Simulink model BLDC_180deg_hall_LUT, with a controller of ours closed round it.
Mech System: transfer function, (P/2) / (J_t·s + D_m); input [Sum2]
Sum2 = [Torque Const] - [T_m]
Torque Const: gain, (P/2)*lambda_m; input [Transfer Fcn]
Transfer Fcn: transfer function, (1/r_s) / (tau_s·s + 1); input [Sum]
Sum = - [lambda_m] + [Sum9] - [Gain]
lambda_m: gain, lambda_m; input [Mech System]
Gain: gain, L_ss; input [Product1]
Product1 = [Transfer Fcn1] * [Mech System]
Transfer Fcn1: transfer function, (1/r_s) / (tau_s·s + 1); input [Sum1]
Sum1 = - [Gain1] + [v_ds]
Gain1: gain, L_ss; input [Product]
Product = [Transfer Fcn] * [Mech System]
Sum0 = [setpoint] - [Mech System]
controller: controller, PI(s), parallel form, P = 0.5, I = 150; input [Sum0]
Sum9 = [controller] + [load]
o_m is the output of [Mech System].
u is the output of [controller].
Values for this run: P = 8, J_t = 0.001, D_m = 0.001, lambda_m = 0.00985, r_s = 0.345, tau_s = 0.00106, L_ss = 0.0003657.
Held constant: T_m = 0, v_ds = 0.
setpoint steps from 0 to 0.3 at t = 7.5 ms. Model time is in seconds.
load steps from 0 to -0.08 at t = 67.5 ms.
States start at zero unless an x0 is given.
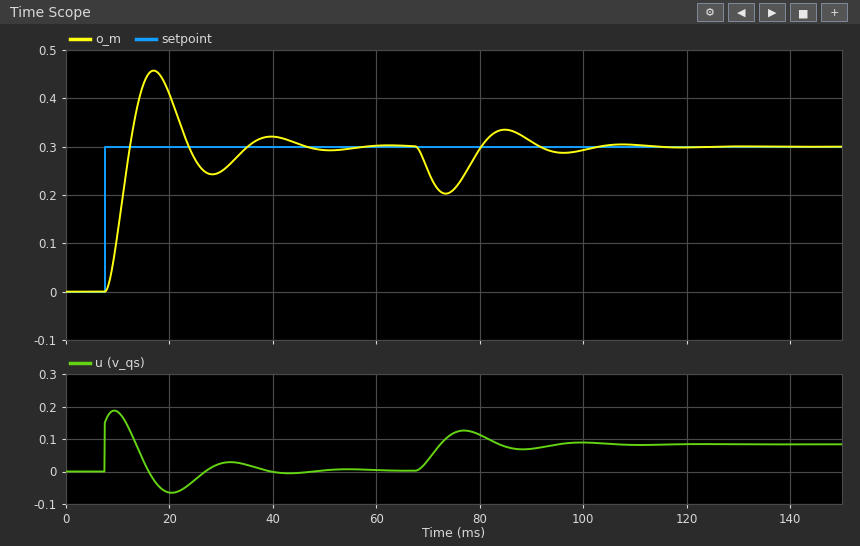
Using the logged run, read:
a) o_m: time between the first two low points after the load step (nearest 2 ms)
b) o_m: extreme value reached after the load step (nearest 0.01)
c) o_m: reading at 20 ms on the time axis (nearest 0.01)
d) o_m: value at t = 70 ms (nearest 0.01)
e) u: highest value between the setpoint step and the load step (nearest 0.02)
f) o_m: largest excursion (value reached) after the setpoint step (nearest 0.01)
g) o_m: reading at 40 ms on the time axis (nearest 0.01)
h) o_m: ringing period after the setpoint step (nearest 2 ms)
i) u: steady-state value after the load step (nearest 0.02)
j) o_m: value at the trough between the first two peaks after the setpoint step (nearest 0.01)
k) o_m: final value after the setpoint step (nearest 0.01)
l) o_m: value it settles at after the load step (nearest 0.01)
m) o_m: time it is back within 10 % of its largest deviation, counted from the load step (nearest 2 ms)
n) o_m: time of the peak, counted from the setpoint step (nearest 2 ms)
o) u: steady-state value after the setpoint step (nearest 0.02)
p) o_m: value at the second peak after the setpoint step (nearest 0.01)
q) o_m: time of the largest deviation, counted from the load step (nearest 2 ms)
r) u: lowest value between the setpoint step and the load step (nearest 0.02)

22 ms
0.20
0.41
0.25
0.18
0.46
0.32
22 ms
0.08
0.24
0.30
0.30
32 ms
10 ms
0.00
0.32
6 ms
-0.06
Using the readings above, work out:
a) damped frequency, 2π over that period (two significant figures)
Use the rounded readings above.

0.29 rad/ms
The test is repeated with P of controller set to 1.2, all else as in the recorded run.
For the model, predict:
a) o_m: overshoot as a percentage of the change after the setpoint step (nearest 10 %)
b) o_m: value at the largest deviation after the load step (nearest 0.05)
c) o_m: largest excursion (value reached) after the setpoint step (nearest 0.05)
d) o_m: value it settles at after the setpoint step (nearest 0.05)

30 %
0.25
0.40
0.30
